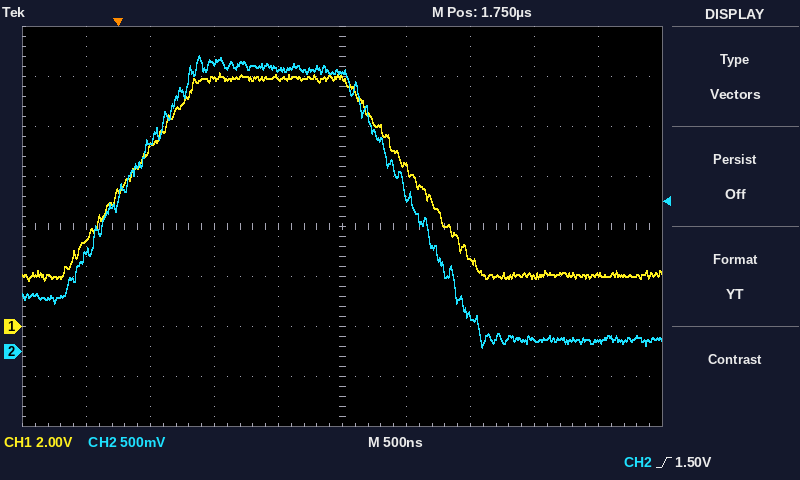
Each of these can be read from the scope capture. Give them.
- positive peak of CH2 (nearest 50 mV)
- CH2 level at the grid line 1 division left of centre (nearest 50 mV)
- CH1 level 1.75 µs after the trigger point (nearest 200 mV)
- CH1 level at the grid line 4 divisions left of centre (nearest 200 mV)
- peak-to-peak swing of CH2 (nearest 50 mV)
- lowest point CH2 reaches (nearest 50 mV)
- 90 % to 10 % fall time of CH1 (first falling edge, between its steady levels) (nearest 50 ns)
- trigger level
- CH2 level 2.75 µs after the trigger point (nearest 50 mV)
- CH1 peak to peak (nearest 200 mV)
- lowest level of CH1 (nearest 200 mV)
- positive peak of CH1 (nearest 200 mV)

2.95 V
2.80 V
10.0 V
3.4 V
2.90 V
50 mV
850 ns
1.50 V
350 mV
8.4 V
1.8 V
10.2 V
